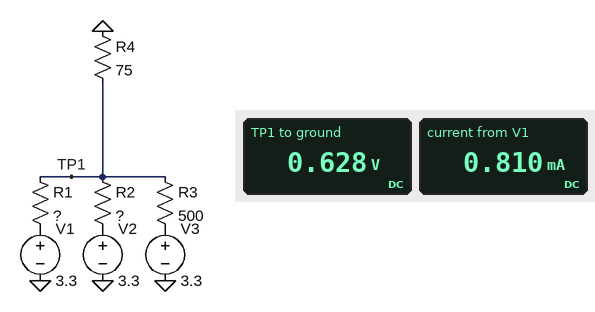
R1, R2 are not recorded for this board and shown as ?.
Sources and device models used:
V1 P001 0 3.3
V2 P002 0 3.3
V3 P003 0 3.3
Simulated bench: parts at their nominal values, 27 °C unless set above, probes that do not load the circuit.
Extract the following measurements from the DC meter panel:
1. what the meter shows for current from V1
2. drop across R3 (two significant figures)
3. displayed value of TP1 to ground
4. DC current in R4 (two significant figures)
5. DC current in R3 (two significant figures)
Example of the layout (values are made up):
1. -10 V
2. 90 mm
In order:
1. 0.810 mA
2. 2.7 V
3. 0.628 V
4. 8.4 mA
5. 5.3 mA
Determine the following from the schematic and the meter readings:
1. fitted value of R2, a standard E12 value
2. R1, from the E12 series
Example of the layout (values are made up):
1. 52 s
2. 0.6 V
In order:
1. 1.2 kΩ
2. 3.3 kΩ
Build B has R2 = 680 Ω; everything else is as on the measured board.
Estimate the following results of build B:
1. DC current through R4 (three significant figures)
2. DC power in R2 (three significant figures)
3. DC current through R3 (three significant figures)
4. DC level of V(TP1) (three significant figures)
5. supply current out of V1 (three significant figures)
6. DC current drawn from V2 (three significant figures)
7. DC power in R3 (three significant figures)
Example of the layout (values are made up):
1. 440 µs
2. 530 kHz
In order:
1. 9.71 mA
2. 9.73 mW
3. 5.14 mA
4. 728 mV
5. 779 µA
6. 3.78 mA
7. 13.2 mW
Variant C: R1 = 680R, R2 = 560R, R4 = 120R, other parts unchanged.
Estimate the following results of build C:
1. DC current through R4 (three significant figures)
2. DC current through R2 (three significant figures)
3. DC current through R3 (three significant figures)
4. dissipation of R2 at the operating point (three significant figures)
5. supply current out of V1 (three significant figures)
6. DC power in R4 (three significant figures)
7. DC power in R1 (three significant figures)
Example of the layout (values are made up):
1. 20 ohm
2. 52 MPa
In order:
1. 10.6 mA
2. 3.61 mA
3. 4.05 mA
4. 7.31 mW
5. 2.98 mA
6. 13.6 mW
7. 6.02 mW
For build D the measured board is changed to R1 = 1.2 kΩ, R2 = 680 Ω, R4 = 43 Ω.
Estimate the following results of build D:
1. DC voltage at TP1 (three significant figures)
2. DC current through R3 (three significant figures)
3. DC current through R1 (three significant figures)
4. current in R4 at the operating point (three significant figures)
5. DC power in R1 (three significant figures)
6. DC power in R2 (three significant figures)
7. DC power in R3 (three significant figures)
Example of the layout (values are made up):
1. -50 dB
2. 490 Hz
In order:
1. 515 mV
2. 5.57 mA
3. 2.32 mA
4. 12.0 mA
5. 6.46 mW
6. 11.4 mW
7. 15.5 mW
